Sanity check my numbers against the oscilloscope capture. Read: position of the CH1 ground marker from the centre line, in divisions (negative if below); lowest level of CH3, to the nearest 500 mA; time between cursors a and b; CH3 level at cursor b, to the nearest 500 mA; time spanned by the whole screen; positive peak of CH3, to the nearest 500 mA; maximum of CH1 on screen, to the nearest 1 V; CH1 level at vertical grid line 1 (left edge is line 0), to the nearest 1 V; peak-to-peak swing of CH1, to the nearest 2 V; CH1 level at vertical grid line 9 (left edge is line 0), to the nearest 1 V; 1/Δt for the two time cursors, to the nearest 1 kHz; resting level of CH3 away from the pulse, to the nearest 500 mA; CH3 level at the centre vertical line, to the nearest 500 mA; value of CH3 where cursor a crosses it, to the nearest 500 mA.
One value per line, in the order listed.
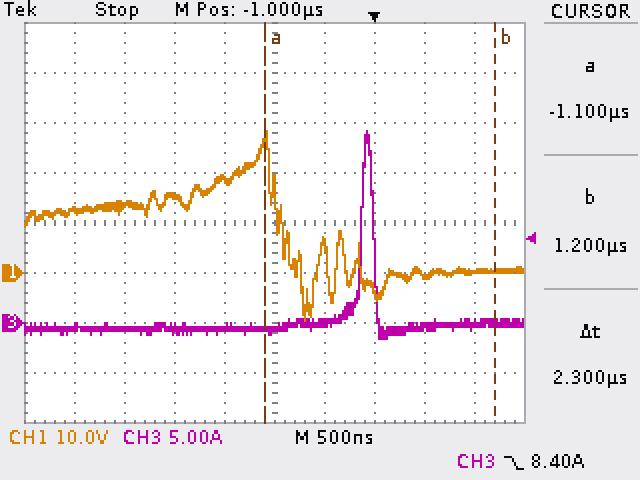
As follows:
-1.0 div
-1.5 A
2.3 µs
0.0 A
5 µs
19.0 A
28 V
12 V
38 V
0 V
435 kHz
-500 mA
-1.0 A
-1.0 A
